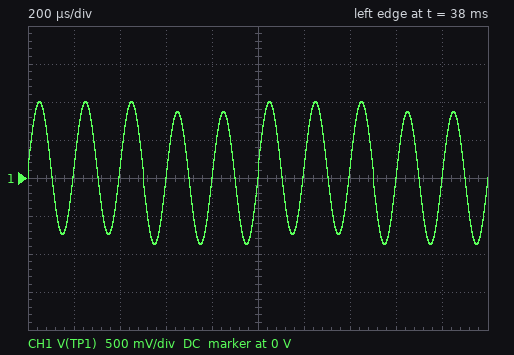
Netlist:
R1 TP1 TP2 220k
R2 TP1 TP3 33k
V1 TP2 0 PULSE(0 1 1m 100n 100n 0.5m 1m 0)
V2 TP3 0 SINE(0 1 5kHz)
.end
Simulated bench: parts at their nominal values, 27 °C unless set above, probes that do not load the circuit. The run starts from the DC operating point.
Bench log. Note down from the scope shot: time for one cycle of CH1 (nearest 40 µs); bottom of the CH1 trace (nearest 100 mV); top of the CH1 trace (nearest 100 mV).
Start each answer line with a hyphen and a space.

- 200 µs
- -900 mV
- 1.0 V
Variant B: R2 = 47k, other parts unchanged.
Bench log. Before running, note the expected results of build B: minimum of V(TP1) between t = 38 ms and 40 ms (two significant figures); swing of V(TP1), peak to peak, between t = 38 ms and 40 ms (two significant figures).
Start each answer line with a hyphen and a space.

- -820 mV
- 1.8 V
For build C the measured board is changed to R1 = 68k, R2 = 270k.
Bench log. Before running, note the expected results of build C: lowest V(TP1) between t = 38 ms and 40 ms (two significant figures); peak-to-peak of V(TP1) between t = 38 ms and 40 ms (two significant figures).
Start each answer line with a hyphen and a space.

- -200 mV
- 1.2 V
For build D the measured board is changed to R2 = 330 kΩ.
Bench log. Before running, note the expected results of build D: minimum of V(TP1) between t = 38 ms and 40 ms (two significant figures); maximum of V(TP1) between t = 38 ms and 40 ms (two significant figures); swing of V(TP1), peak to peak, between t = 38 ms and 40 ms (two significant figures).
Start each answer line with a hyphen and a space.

- -400 mV
- 1.0 V
- 1.4 V
